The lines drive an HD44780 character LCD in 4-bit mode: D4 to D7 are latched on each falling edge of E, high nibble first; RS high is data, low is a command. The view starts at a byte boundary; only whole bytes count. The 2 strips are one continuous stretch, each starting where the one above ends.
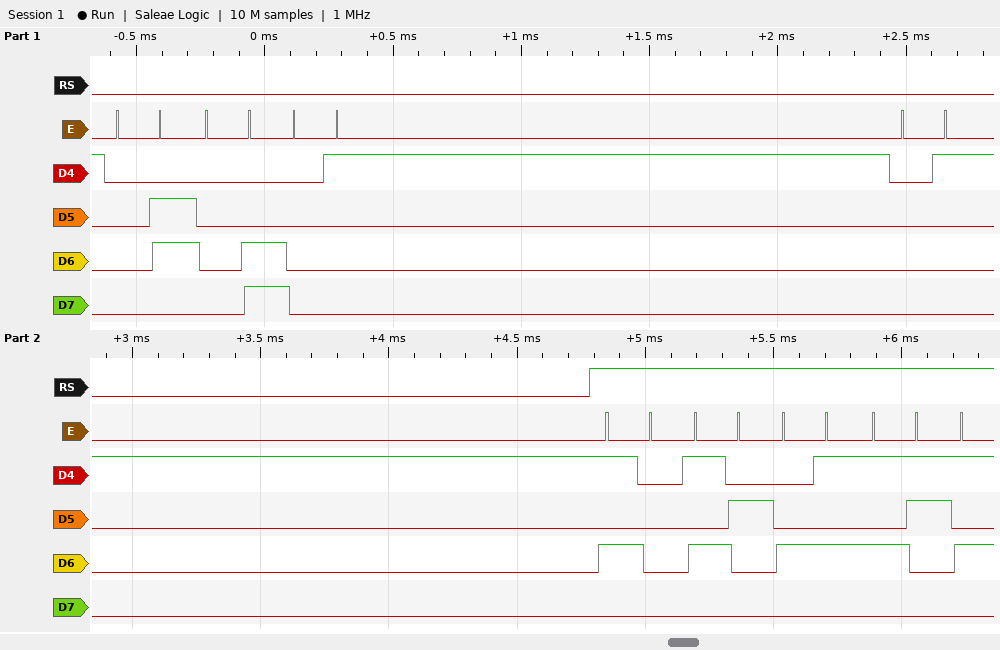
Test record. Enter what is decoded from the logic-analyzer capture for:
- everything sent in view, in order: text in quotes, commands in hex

0x06 0x0C 0x01 0x01 "PRES"
